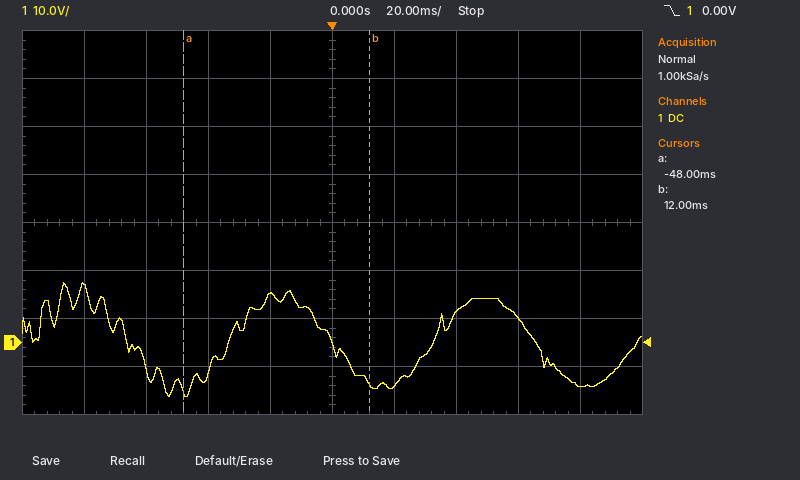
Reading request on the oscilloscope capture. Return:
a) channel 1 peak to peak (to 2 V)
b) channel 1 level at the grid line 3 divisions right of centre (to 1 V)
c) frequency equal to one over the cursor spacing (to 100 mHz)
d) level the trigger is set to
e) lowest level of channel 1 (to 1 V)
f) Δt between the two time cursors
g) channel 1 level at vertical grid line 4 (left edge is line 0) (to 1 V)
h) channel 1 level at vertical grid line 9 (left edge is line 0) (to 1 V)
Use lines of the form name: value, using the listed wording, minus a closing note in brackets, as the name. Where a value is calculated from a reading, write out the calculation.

channel 1 peak to peak: 24 V
channel 1 level at the grid line 3 divisions right of centre: 5 V
frequency equal to one over the cursor spacing: 1 / 60 ms ≈ 16.7 Hz
level the trigger is set to: 0.00 V
lowest level of channel 1: -11 V
Δt between the two time cursors: 12 ms − (-48 ms) = 60 ms
channel 1 level at vertical grid line 4 (left edge is line 0): 10 V
channel 1 level at vertical grid line 9 (left edge is line 0): -9 V
